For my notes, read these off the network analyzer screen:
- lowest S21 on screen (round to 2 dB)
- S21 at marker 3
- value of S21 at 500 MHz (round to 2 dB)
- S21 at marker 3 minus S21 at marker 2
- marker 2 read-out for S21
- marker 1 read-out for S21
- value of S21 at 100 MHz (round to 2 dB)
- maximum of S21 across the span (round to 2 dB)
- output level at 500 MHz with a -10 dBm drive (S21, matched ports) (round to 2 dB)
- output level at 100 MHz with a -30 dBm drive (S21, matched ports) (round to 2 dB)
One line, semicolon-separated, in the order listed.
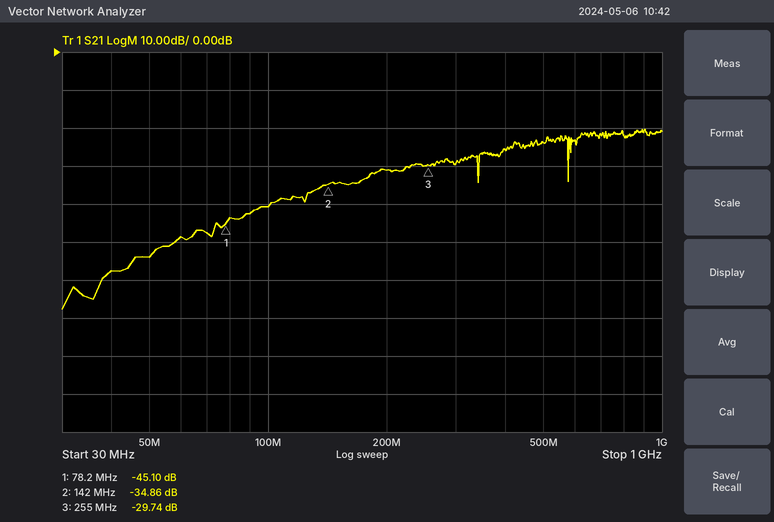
-68 dB; -29.74 dB; -24 dB; 5.12 dB; -34.86 dB; -45.10 dB; -40 dB; -20 dB; -34 dBm; -70 dBm
